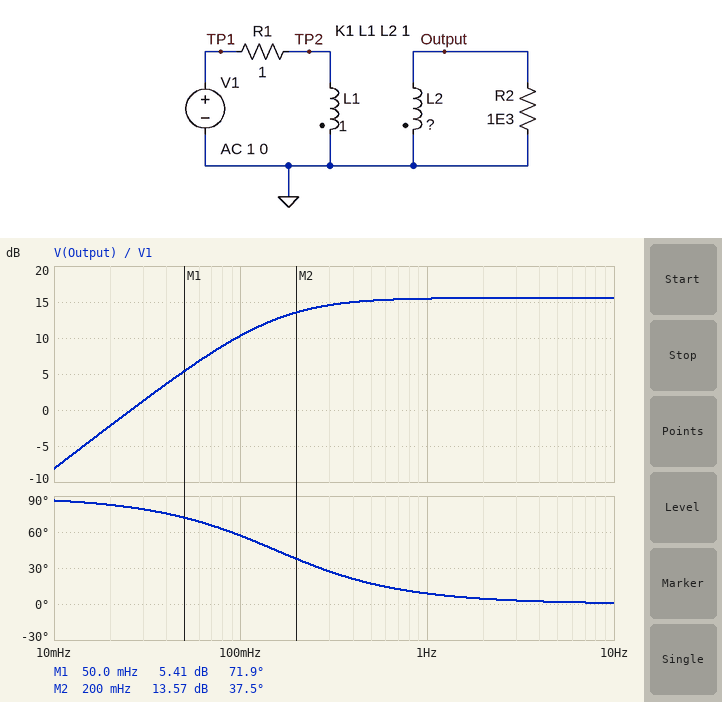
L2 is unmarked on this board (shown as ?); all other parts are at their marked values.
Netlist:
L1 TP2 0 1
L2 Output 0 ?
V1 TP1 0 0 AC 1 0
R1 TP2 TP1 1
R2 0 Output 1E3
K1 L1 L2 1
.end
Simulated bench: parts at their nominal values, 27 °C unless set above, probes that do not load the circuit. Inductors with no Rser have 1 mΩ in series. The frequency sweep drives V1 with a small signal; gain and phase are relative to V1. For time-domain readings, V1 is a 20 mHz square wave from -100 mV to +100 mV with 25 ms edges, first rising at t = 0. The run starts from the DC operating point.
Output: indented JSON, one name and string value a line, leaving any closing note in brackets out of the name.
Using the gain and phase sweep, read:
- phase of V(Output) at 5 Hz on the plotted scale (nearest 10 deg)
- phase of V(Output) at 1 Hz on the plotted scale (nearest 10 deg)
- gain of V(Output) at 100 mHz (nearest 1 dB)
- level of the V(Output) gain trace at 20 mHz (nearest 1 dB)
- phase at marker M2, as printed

{
  "phase of V(Output) at 5 Hz on the plotted scale": "0 deg",
  "phase of V(Output) at 1 Hz on the plotted scale": "10 deg",
  "gain of V(Output) at 100 mHz": "10 dB",
  "level of the V(Output) gain trace at 20 mHz": "-2 dB",
  "phase at marker M2, as printed": "37.5 deg"
}
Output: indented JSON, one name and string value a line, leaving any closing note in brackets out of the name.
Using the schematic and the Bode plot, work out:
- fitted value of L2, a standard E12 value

{
  "fitted value of L2, a standard E12 value": "39 H"
}
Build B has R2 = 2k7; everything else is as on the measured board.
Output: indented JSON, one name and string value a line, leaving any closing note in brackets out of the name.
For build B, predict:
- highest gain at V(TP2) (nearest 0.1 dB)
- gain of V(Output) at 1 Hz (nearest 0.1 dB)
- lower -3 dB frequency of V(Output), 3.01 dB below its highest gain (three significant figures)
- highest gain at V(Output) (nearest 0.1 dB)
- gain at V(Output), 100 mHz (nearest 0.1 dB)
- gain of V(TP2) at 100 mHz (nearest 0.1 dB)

{
  "highest gain at V(TP2)": "-0.1 dB",
  "gain of V(Output) at 1 Hz": "15.7 dB",
  "lower -3 dB frequency of V(Output), 3.01 dB below its highest gain": "157 mHz",
  "highest gain at V(Output)": "15.8 dB",
  "gain at V(Output), 100 mHz": "10.4 dB",
  "gain of V(TP2) at 100 mHz": "-5.5 dB"
}
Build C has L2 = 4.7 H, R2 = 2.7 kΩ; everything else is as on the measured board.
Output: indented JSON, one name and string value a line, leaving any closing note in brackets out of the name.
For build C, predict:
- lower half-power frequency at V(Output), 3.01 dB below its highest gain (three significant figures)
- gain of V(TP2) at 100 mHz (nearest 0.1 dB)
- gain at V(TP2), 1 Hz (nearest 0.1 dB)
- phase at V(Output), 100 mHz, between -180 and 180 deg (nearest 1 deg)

{
  "lower half-power frequency at V(Output), 3.01 dB below its highest gain": "159 mHz",
  "gain of V(TP2) at 100 mHz": "-5.5 dB",
  "gain at V(TP2), 1 Hz": "-0.1 dB",
  "phase at V(Output), 100 mHz, between -180 and 180 deg": "58 deg"
}
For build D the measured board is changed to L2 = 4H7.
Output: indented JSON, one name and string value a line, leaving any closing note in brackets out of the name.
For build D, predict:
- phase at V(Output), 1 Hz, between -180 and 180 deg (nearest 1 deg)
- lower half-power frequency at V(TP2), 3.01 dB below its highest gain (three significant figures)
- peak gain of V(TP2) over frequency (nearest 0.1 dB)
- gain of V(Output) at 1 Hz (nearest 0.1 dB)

{
  "phase at V(Output), 1 Hz, between -180 and 180 deg": "9 deg",
  "lower half-power frequency at V(TP2), 3.01 dB below its highest gain": "159 mHz",
  "peak gain of V(TP2) over frequency": "0 dB",
  "gain of V(Output) at 1 Hz": "6.6 dB"
}
